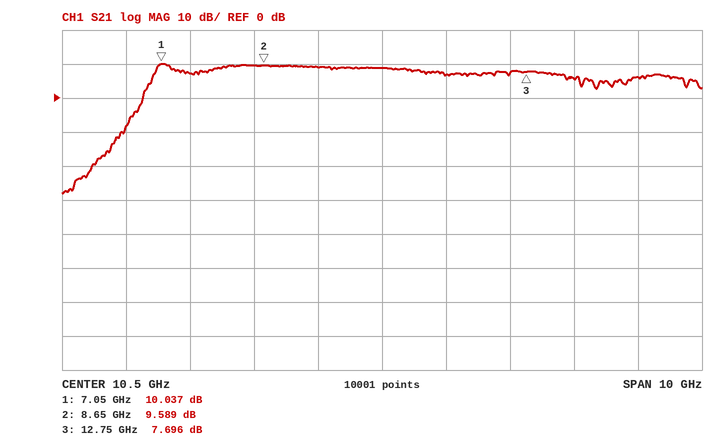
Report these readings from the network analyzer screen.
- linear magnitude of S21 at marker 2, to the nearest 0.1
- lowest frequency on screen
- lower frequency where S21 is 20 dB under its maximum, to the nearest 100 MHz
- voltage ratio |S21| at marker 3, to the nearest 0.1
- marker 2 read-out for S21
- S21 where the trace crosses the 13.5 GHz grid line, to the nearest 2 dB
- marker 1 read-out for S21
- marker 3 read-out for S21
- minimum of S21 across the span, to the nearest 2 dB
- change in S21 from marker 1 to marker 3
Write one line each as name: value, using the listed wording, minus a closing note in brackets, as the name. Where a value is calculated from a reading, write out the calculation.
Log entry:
linear magnitude of S21 at marker 2, to the nearest 0.1: 10^(9.589/20) ≈ 3.0
lowest frequency on screen: 5.5 GHz
lower frequency where S21 is 20 dB under its maximum, to the nearest 100 MHz: 6.5 GHz
voltage ratio |S21| at marker 3, to the nearest 0.1: 10^(7.696/20) ≈ 2.4
marker 2 read-out for S21: 9.589 dB
S21 where the trace crosses the 13.5 GHz grid line, to the nearest 2 dB: 6 dB
marker 1 read-out for S21: 10.037 dB
marker 3 read-out for S21: 7.696 dB
minimum of S21 across the span, to the nearest 2 dB: -28 dB
change in S21 from marker 1 to marker 3: 7.696 − (10.037) = -2.341 dB
